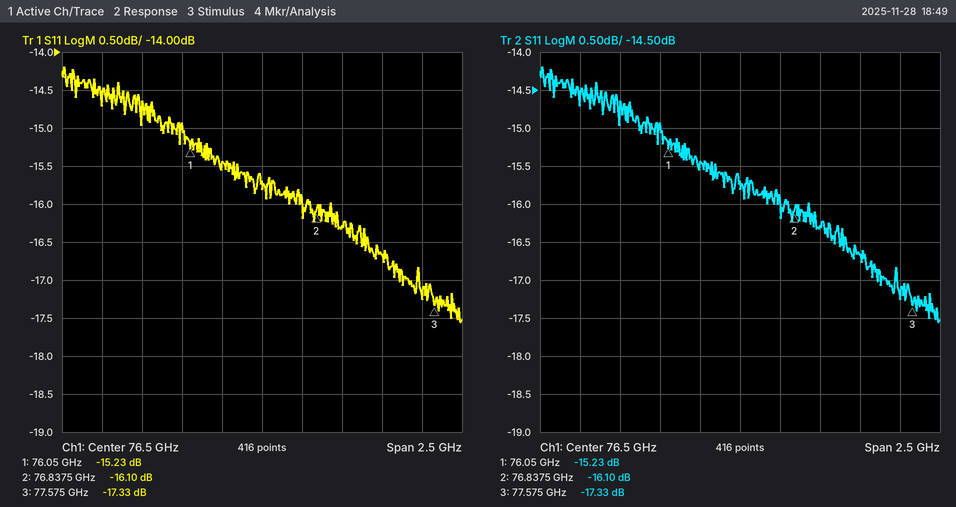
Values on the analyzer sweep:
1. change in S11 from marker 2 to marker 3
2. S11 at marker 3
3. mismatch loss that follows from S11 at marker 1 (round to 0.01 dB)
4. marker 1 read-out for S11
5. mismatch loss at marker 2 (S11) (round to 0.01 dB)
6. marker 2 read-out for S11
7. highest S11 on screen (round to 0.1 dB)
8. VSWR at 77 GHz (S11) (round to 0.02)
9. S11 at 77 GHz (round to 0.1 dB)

-1.23 dB
-17.33 dB
0.13 dB
-15.23 dB
0.11 dB
-16.10 dB
-14.2 dB
1.36
-16.3 dB
